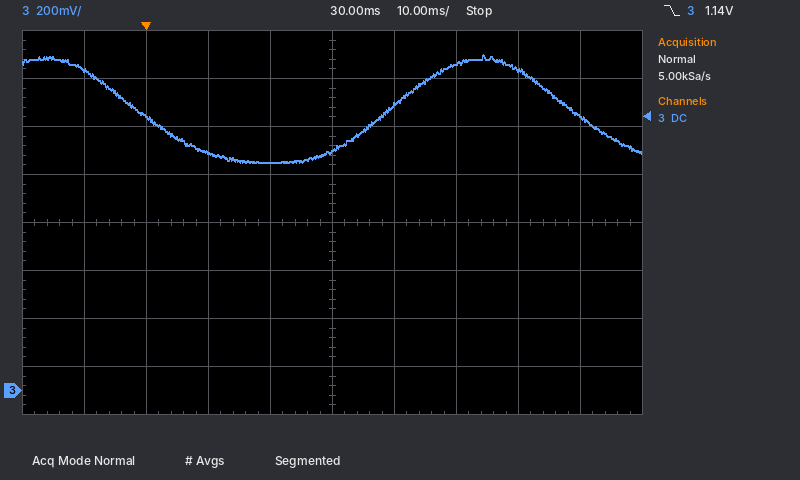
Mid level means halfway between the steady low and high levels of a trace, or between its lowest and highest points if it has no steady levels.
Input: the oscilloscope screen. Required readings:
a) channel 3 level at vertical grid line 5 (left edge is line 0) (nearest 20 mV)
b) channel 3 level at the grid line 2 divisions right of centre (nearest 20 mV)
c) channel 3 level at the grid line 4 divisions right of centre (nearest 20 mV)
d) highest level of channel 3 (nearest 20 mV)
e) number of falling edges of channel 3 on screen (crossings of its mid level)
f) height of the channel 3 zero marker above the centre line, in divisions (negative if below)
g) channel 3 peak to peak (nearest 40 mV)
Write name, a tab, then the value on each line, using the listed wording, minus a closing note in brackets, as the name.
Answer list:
channel 3 level at vertical grid line 5 (left edge is line 0)	1.00 V
channel 3 level at the grid line 2 divisions right of centre	1.36 V
channel 3 level at the grid line 4 divisions right of centre	1.14 V
highest level of channel 3	1.40 V
number of falling edges of channel 3 on screen	2
height of the channel 3 zero marker above the centre line, in divisions	-3.5 div
channel 3 peak to peak	440 mV
